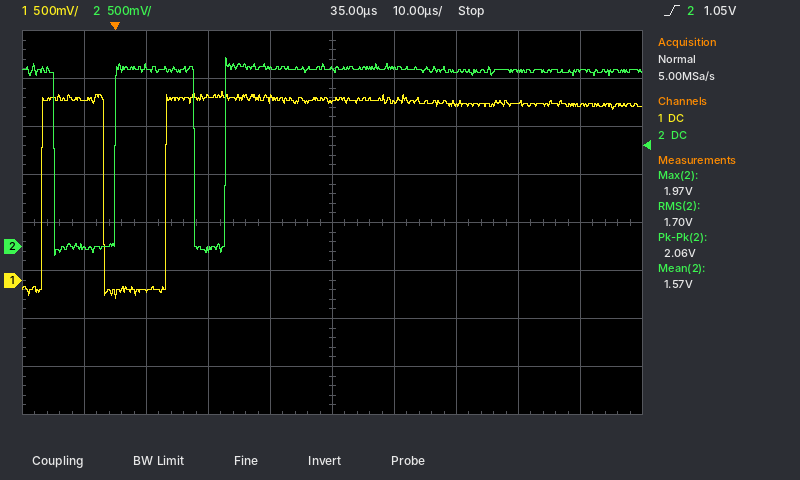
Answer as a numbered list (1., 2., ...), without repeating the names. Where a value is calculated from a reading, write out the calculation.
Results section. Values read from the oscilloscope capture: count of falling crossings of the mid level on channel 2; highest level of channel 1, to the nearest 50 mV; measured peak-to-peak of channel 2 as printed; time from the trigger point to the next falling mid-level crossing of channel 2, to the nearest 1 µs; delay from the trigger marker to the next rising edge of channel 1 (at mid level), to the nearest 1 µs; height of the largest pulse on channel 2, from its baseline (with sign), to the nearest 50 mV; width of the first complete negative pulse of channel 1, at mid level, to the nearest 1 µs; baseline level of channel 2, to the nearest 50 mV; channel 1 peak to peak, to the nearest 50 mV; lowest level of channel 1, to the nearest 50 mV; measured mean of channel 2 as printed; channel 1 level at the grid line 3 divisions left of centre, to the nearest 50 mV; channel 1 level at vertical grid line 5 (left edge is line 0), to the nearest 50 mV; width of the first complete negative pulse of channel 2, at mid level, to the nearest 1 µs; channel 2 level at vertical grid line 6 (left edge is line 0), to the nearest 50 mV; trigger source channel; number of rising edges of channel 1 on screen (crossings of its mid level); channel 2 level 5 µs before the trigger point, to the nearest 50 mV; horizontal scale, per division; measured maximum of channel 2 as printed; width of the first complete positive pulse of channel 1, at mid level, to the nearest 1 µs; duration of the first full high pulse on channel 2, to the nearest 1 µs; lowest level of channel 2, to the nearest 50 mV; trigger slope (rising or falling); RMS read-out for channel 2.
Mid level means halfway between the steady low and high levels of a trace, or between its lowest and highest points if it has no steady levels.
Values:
1. 2
2. 1.95 V
3. 2.06 V
4. 13 µs
5. 8 µs
6. -100 mV − (1.85 V) = -1.95 V
7. 10 µs
8. 1.85 V
9. 1.95 V − (-200 mV) = 2.15 V
10. -200 mV
11. 1.57 V
12. -100 mV
13. 1.85 V
14. 10 µs
15. 1.85 V
16. channel 2
17. 2
18. 0 mV
19. 10 µs
20. 1.97 V
21. 10 µs
22. 13 µs
23. -100 mV
24. rising
25. 1.70 V
